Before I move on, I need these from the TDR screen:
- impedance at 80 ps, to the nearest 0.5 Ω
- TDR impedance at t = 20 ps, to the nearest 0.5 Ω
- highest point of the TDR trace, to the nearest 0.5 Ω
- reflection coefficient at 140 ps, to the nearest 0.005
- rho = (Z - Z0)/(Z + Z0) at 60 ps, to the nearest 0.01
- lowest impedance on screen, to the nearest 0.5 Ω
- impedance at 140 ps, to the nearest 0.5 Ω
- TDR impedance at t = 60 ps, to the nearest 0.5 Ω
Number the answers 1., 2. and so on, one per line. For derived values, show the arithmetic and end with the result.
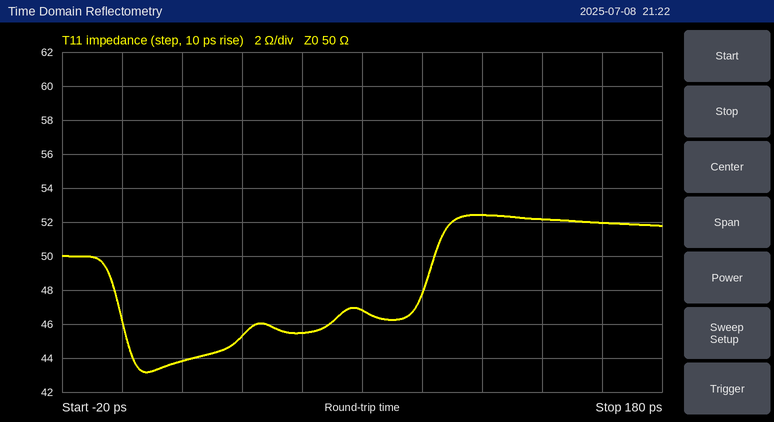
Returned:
1. 47.0 Ω
2. 44.0 Ω
3. 52.5 Ω
4. (52 − 50)/(52 + 50) ≈ +0.020
5. (45.5 − 50)/(45.5 + 50) ≈ -0.05
6. 43.0 Ω
7. 52.0 Ω
8. 45.5 Ω
